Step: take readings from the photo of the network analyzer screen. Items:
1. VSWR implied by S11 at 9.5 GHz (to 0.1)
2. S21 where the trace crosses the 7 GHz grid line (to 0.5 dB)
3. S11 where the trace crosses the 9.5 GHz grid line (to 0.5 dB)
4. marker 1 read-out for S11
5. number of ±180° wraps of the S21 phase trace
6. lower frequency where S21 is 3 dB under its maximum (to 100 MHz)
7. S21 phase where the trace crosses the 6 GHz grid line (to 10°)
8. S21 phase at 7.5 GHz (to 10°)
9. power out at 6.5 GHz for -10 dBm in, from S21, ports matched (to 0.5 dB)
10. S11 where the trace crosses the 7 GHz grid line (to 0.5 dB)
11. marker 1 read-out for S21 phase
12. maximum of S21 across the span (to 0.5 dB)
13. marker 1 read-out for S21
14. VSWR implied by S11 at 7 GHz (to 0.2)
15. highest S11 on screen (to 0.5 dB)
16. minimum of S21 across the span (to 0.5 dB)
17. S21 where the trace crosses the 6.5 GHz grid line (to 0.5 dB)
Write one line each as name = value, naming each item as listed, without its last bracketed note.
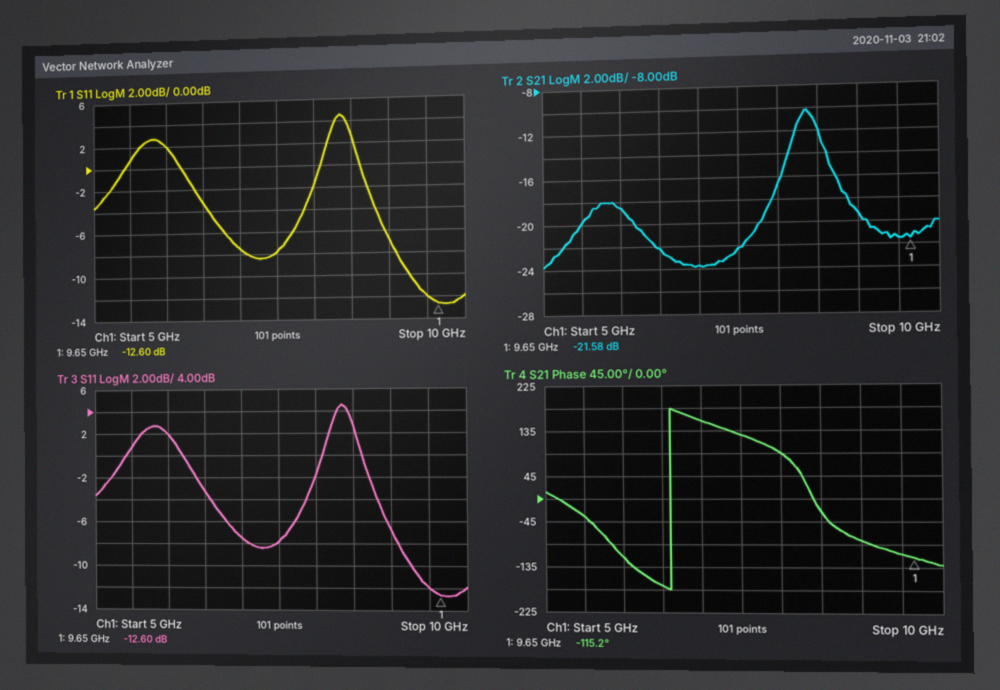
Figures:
VSWR implied by S11 at 9.5 GHz = 1.7
S21 where the trace crosses the 7 GHz grid line = -23.5 dB
S11 where the trace crosses the 9.5 GHz grid line = -12.0 dB
marker 1 read-out for S11 = -12.60 dB
number of ±180° wraps of the S21 phase trace = 1
lower frequency where S21 is 3 dB under its maximum = 8.2 GHz
S21 phase where the trace crosses the 6 GHz grid line = -120°
S21 phase at 7.5 GHz = 130°
power out at 6.5 GHz for -10 dBm in, from S21, ports matched = -32.0 dBm
S11 where the trace crosses the 7 GHz grid line = -7.5 dB
marker 1 read-out for S21 phase = -115.2°
maximum of S21 across the span = -10.0 dB
marker 1 read-out for S21 = -21.58 dB
VSWR implied by S11 at 7 GHz = 2.4
highest S11 on screen = 4.5 dB
minimum of S21 across the span = -24.0 dB
S21 where the trace crosses the 6.5 GHz grid line = -22.0 dB
